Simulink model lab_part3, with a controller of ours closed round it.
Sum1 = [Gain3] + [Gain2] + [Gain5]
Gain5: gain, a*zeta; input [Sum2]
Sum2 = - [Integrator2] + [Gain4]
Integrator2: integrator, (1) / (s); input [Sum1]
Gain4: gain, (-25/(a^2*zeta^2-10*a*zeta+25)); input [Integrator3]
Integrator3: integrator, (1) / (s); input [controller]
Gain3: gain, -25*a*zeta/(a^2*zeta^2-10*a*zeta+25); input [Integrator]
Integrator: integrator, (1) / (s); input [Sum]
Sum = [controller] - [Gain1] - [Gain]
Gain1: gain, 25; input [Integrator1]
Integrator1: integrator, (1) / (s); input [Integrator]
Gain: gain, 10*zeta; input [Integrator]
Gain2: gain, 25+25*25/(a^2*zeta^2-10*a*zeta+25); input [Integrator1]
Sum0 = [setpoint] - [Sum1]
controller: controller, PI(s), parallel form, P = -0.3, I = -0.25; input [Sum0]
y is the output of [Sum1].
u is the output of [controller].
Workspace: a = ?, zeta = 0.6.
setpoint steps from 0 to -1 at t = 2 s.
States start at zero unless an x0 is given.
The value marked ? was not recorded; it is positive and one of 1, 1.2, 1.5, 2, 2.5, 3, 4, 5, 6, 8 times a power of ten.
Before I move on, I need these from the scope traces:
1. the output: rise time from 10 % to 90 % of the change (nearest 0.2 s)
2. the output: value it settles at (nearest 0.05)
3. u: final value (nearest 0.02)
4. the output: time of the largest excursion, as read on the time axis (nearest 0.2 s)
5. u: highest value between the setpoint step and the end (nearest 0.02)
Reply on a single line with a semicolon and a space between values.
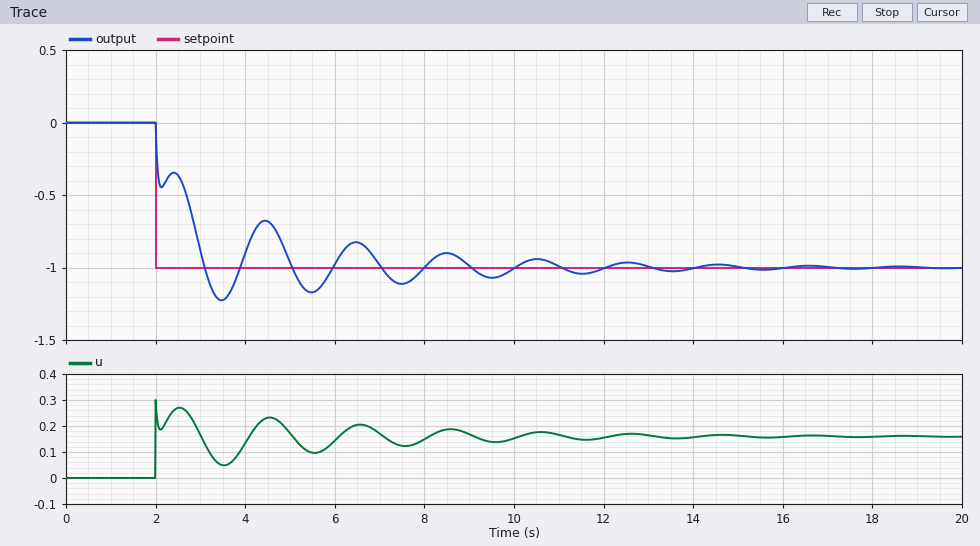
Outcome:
1.0 s; -1.00; 0.16; 3.4 s; 0.30
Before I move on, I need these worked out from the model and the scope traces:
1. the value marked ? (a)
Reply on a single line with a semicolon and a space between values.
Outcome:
5
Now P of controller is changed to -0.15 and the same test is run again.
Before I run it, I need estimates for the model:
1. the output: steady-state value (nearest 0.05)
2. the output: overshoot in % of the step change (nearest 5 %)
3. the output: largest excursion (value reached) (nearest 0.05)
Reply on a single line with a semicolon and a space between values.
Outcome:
-1.00; 15 %; -1.15
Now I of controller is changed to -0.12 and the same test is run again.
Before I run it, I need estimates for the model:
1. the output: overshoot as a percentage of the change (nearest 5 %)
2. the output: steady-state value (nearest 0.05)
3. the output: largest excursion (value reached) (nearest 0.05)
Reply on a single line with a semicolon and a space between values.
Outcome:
10 %; -1.00; -1.10
